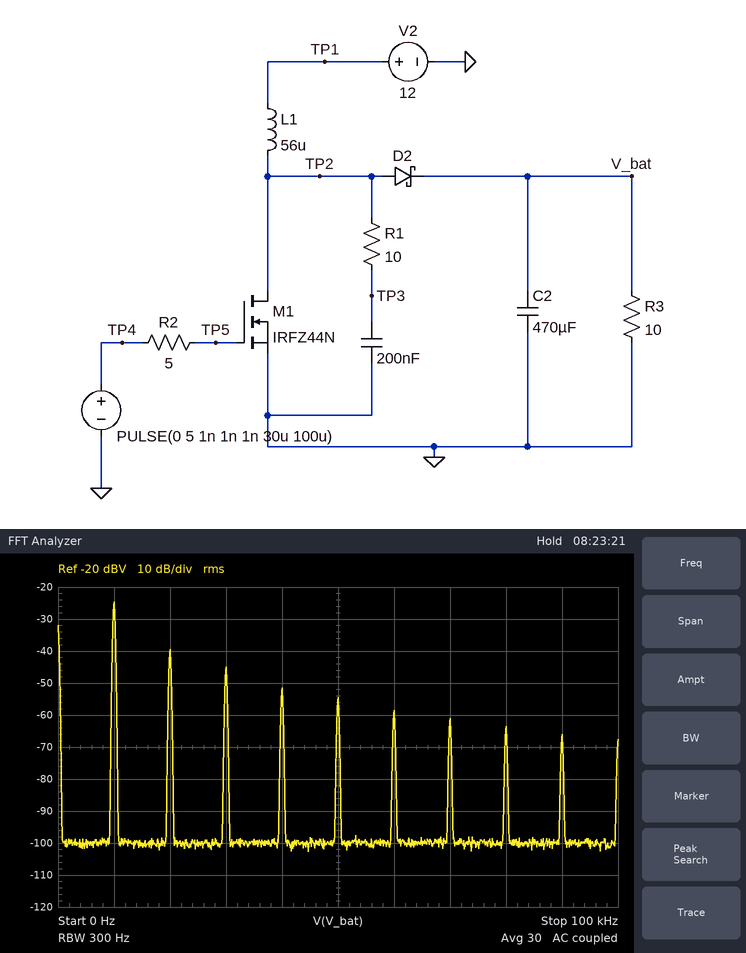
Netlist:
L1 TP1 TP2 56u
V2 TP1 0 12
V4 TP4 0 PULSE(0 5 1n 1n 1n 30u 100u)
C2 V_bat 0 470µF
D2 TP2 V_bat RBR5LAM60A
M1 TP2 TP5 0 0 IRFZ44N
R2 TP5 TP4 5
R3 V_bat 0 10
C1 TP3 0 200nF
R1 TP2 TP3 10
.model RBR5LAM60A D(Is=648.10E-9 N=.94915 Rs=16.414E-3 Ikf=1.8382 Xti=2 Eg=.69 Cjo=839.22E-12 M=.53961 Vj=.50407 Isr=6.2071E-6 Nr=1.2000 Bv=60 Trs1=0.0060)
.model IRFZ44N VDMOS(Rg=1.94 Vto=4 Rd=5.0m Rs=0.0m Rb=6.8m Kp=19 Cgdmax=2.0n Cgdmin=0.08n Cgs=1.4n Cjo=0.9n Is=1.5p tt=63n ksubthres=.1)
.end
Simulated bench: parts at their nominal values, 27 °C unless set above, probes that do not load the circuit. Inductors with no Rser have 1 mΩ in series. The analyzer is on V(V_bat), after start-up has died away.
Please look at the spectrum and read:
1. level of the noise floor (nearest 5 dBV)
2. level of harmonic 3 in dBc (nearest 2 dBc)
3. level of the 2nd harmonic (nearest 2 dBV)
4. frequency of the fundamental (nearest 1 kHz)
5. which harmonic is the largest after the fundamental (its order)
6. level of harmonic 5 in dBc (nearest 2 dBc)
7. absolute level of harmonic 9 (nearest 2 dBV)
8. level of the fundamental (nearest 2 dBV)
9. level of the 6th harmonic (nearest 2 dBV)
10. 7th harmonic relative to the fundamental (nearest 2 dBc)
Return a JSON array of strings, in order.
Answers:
["-100 dBV", "-20 dBc", "-40 dBV", "10 kHz", "2", "-30 dBc", "-66 dBV", "-24 dBV", "-58 dBV", "-36 dBc"]
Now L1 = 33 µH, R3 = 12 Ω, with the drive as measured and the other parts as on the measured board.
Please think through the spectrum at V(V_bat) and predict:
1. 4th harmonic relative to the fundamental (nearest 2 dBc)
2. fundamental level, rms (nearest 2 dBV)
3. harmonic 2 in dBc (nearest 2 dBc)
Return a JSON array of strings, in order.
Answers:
["-24 dBc", "-22 dBV", "-10 dBc"]
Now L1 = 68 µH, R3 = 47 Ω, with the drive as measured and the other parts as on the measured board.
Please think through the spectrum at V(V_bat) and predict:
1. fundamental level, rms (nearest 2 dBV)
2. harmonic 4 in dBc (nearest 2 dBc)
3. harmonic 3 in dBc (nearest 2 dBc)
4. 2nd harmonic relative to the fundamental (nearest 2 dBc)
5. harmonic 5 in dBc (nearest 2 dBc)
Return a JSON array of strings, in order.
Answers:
["-32 dBV", "-20 dBc", "-14 dBc", "-8 dBc", "-26 dBc"]
